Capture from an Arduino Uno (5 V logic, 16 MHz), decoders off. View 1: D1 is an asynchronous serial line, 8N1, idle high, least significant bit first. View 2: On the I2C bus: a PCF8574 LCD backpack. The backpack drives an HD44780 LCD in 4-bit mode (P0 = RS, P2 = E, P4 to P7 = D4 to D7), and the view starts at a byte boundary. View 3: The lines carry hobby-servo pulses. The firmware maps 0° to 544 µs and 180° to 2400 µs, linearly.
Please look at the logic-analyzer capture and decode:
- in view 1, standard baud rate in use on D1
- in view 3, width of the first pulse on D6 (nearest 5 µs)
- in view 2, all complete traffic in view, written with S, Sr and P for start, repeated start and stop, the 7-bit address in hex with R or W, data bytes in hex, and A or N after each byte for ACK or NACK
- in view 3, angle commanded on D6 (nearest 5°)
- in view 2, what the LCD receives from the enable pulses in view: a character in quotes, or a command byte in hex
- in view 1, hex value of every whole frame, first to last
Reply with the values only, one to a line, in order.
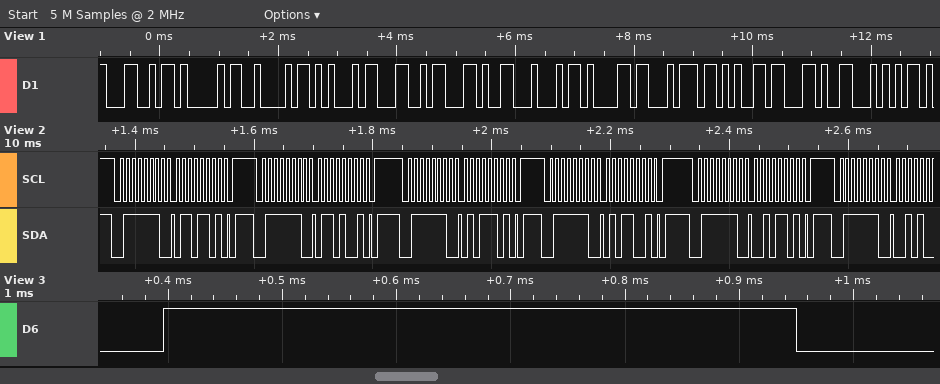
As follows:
9600 baud
555 µs
S 3FW A 6D A P S 3FW A 69 A P S 3FW A 5D A P S 3FW A 59 A P S 3FW A 2D A P S 3FW A
0°
'e'
0x4C 0x41 0x42 0x45 0x4C 0x2C 0x44 0x61 0x74 0x65 0x2C 0x54
